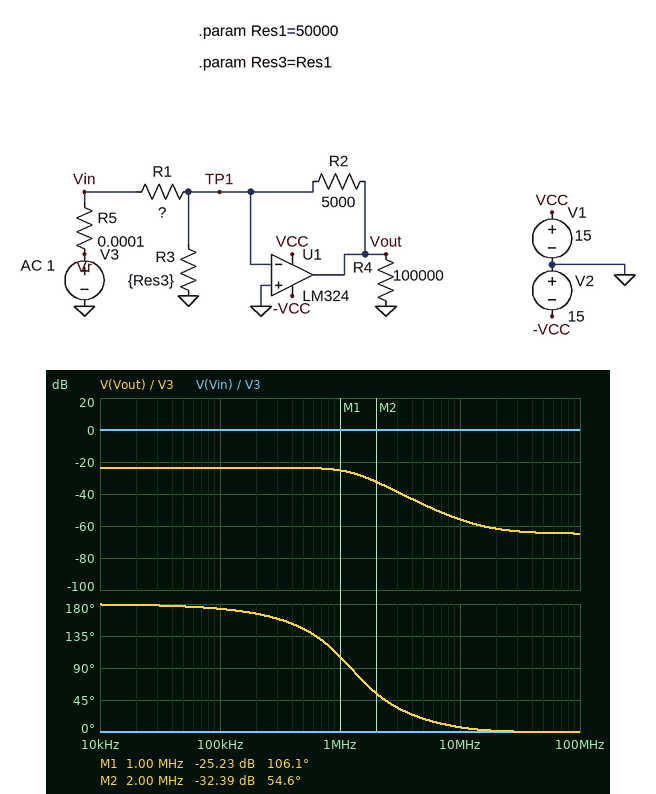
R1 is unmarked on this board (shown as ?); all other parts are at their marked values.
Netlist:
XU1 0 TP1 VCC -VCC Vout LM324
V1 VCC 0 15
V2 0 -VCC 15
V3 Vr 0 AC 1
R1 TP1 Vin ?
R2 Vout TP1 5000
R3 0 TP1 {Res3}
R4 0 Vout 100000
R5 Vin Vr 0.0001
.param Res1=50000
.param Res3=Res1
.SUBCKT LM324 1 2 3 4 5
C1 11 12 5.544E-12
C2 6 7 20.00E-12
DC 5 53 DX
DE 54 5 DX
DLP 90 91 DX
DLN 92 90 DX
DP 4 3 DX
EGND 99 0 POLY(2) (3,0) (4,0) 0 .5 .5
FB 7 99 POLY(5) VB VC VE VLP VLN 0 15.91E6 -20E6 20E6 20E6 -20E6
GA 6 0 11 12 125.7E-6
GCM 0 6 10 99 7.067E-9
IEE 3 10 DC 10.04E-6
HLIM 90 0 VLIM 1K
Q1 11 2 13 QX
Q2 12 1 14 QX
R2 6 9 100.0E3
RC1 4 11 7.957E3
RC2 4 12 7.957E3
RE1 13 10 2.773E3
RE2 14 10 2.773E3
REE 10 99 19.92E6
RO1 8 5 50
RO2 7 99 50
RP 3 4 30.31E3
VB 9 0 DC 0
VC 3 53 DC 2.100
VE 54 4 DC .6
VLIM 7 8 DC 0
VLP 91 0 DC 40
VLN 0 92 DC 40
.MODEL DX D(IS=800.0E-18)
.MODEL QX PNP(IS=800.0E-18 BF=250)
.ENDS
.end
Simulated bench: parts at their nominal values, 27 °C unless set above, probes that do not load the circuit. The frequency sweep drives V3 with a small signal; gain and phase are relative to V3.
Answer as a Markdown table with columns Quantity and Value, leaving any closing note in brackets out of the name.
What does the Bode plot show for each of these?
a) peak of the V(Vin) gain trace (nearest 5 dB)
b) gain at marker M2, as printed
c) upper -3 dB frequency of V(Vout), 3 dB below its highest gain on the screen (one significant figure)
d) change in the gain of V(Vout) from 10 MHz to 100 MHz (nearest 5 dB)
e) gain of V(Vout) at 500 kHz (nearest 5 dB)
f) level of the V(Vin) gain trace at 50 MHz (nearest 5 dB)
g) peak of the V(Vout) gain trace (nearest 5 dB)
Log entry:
| Quantity | Value |
|---|---|
| peak of the V(Vin) gain trace | 0 dB |
| gain at marker M2, as printed | -32.39 dB |
| upper -3 dB frequency of V(Vout), 3 dB below its highest gain on the screen | 1 MHz |
| change in the gain of V(Vout) from 10 MHz to 100 MHz | -10 dB |
| gain of V(Vout) at 500 kHz | -25 dB |
| level of the V(Vin) gain trace at 50 MHz | 0 dB |
| peak of the V(Vout) gain trace | -25 dB |
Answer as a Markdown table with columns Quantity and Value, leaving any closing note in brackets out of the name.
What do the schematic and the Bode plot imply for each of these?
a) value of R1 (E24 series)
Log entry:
| Quantity | Value |
|---|---|
| value of R1 | 75 kΩ |
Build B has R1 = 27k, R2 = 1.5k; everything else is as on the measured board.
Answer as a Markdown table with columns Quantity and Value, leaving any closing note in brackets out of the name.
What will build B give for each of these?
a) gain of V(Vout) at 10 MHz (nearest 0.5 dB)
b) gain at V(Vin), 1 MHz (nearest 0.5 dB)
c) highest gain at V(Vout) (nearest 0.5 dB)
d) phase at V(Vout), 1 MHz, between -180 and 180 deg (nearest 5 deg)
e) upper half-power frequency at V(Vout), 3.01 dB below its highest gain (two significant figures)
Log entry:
| Quantity | Value |
|---|---|
| gain of V(Vout) at 10 MHz | -51.5 dB |
| gain at V(Vin), 1 MHz | 0 dB |
| highest gain at V(Vout) | -25.0 dB |
| phase at V(Vout), 1 MHz, between -180 and 180 deg | 110 deg |
| upper half-power frequency at V(Vout), 3.01 dB below its highest gain | 1.3 MHz |
